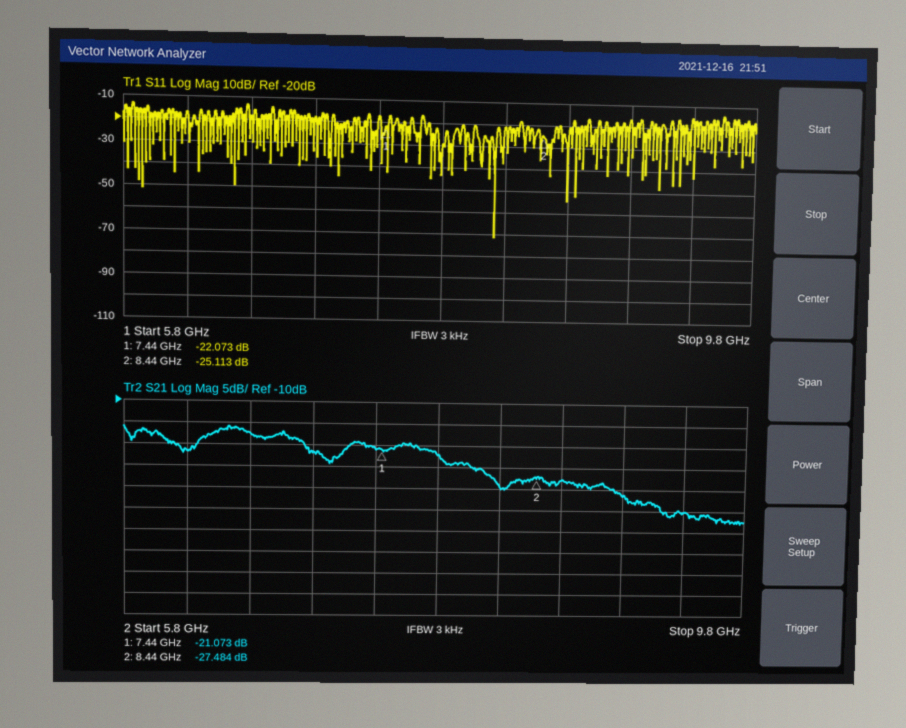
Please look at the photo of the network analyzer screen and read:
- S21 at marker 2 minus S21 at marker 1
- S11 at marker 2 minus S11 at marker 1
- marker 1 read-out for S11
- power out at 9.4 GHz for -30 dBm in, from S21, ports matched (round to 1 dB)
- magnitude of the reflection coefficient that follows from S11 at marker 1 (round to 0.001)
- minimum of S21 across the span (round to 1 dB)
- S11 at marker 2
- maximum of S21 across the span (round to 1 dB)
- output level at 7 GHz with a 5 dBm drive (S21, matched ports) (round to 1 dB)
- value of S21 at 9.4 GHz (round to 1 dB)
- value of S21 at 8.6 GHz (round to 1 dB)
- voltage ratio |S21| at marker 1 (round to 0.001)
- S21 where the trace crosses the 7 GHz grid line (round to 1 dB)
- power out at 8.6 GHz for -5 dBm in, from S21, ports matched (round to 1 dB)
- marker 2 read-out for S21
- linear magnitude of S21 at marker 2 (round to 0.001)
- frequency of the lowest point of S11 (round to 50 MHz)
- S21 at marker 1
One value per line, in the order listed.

-6.411 dB
-3.040 dB
-22.073 dB
-65 dBm
0.079
-38 dB
-25.113 dB
-16 dB
-17 dBm
-35 dB
-28 dB
0.088
-22 dB
-33 dBm
-27.484 dB
0.042
8.15 GHz
-21.073 dB
